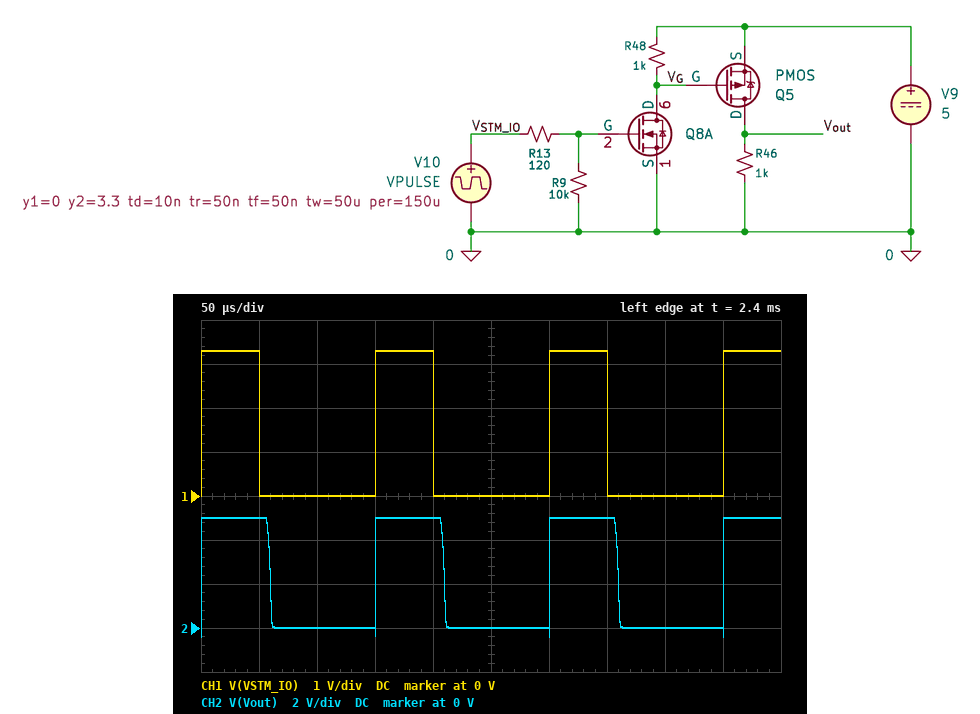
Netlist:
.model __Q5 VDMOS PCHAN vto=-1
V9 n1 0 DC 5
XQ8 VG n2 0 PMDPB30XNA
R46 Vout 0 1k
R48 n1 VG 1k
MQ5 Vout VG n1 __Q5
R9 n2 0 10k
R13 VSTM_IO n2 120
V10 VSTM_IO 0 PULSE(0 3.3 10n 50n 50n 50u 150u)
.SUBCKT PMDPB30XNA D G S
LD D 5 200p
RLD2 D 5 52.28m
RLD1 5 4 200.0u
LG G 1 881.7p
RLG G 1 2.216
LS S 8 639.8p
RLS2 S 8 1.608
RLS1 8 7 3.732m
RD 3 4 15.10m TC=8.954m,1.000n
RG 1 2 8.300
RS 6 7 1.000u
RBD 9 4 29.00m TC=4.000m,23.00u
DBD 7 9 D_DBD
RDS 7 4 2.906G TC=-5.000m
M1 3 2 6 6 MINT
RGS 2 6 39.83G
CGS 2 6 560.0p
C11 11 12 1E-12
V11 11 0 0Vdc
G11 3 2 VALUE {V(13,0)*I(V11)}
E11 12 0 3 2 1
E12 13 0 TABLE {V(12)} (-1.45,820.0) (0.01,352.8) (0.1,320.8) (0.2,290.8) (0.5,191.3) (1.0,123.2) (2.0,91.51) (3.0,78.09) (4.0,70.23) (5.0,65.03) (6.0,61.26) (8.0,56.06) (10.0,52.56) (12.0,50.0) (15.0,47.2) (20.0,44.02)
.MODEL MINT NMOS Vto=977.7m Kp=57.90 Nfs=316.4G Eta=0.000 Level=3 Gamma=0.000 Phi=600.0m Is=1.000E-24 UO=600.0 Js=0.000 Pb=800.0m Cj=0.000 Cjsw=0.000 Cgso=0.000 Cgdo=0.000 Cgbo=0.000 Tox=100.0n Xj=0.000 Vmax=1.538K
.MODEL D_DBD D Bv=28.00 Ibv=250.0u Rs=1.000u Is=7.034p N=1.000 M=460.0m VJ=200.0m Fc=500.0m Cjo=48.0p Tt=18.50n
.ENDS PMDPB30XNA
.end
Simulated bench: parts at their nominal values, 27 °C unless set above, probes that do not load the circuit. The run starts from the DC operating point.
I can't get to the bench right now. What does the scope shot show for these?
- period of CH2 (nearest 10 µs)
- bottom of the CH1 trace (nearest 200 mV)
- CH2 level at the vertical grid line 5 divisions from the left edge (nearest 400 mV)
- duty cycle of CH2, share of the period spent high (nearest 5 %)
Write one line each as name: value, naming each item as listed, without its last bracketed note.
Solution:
period of CH2: 150 µs
bottom of the CH1 trace: 0 V
CH2 level at the vertical grid line 5 divisions from the left edge: 0 V
duty cycle of CH2, share of the period spent high: 40 %
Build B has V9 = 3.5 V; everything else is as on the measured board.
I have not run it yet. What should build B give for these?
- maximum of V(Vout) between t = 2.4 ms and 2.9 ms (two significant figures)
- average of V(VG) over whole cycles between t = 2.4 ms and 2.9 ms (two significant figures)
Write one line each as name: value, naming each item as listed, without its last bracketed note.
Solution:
maximum of V(Vout) between t = 2.4 ms and 2.9 ms: 3.5 V
average of V(VG) over whole cycles between t = 2.4 ms and 2.9 ms: 2.2 V
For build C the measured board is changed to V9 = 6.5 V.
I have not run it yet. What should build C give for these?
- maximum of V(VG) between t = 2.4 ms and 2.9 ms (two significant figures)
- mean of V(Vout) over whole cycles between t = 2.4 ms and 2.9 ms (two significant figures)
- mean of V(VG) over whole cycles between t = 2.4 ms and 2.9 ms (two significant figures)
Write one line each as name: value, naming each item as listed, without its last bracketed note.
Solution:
maximum of V(VG) between t = 2.4 ms and 2.9 ms: 6.5 V
mean of V(Vout) over whole cycles between t = 2.4 ms and 2.9 ms: 2.6 V
mean of V(VG) over whole cycles between t = 2.4 ms and 2.9 ms: 4.2 V
